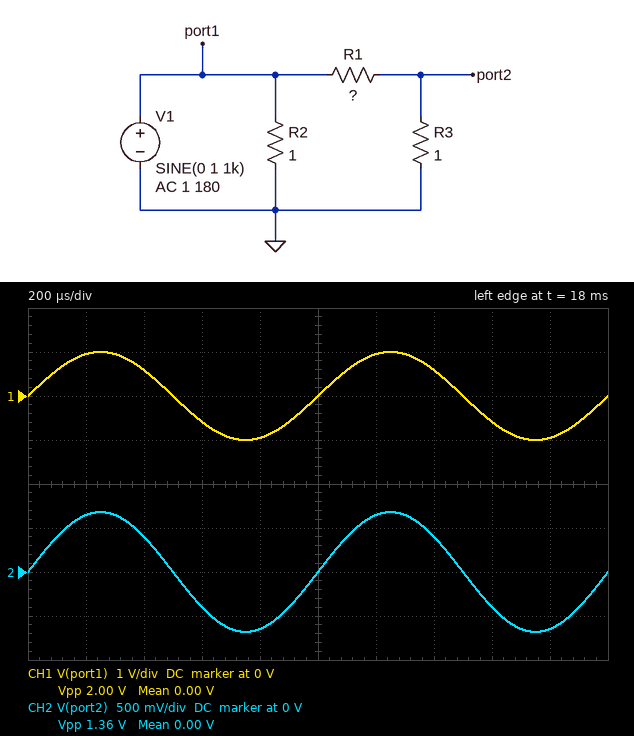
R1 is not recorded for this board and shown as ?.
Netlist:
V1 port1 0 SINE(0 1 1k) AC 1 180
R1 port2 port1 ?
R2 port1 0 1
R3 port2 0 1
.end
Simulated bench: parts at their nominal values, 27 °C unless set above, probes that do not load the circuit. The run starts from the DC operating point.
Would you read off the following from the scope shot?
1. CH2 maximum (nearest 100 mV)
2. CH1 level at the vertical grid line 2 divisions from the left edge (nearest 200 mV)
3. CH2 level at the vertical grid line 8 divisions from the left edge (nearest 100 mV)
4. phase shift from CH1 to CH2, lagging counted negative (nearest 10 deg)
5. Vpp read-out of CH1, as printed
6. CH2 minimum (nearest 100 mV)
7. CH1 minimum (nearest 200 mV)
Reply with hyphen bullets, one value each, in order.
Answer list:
- 700 mV
- 600 mV
- -400 mV
- 0 deg
- 2.00 V
- -700 mV
- -1.0 V
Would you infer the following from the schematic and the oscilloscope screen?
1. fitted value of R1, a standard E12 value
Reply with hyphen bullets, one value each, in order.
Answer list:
- 0.47 Ω
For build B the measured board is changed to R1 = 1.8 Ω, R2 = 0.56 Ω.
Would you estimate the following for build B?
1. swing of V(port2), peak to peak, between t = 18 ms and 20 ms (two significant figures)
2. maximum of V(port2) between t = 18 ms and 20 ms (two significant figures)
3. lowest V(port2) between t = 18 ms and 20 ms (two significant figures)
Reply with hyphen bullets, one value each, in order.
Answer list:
- 710 mV
- 360 mV
- -360 mV
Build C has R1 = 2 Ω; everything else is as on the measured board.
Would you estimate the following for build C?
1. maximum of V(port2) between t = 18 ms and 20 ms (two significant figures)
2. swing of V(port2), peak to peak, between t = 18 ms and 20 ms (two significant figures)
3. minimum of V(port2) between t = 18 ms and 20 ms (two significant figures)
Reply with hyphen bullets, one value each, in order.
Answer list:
- 330 mV
- 670 mV
- -330 mV
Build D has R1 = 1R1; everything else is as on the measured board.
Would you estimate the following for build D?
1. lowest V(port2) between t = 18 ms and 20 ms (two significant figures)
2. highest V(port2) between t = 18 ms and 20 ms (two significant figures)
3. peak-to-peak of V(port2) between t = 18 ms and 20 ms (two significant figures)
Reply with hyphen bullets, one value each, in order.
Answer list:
- -480 mV
- 480 mV
- 950 mV
